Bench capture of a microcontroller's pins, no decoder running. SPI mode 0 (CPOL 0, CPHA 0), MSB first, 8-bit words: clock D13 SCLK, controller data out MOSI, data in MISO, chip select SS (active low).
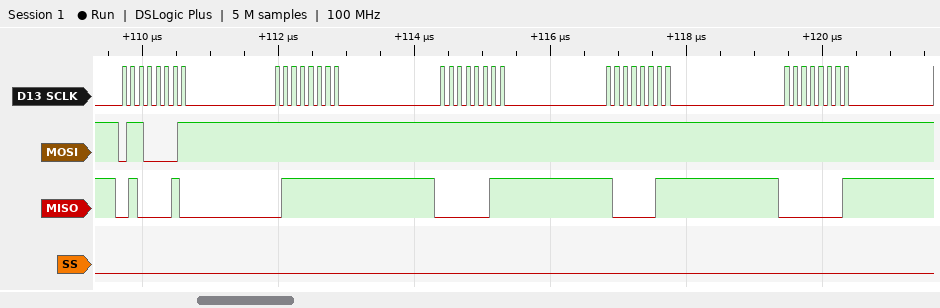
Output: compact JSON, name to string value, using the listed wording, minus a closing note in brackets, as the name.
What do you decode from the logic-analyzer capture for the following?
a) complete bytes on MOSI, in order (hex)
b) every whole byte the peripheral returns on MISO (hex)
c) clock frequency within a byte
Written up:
{"complete bytes on MOSI, in order": "0x61 0xFF 0xFF 0xFF 0xFF", "every whole byte the peripheral returns on MISO": "0x42 0x7F 0x03 0x83 0x01", "clock frequency within a byte": "8 MHz"}
